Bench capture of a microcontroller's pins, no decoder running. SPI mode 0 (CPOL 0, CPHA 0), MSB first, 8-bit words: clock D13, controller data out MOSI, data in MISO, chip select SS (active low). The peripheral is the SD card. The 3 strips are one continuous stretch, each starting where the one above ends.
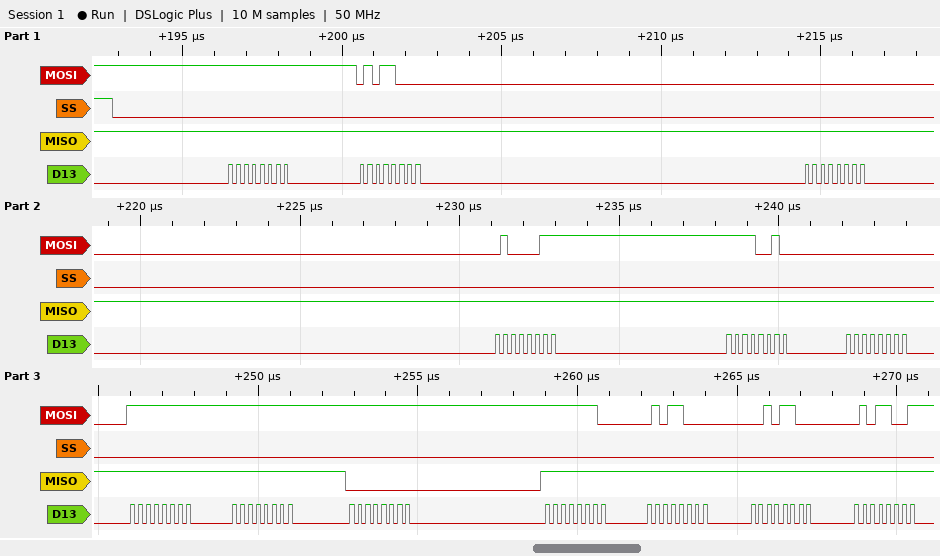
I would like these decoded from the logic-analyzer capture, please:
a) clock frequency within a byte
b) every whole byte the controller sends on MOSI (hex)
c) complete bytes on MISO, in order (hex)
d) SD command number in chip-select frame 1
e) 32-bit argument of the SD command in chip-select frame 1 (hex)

4 MHz
FF 58 00 43 F2 00 FF FF FF FE 58 2C 59
FF FF FF FF FF FF FF FF 00 FF FF FF FF
CMD24
0x0043F200
